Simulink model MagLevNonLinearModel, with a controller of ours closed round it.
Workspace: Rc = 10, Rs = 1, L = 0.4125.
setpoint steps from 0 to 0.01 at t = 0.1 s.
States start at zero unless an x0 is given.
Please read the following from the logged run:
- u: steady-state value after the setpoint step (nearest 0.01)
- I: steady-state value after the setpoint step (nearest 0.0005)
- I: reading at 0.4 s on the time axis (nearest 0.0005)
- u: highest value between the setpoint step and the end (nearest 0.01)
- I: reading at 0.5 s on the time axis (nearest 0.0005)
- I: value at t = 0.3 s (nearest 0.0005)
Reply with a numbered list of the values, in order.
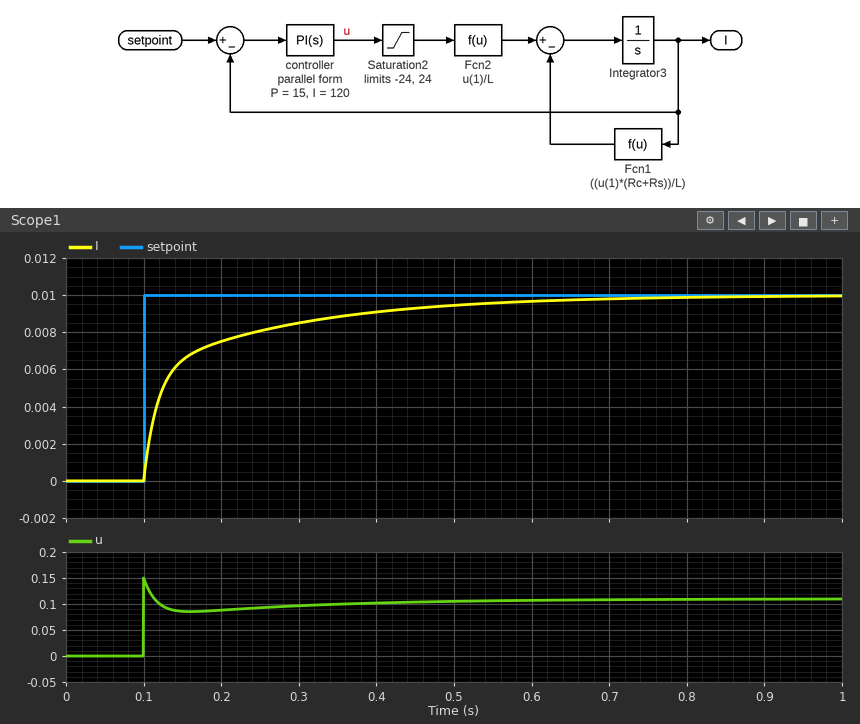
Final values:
1. 0.11
2. 0.0100
3. 0.0090
4. 0.15
5. 0.0095
6. 0.0085
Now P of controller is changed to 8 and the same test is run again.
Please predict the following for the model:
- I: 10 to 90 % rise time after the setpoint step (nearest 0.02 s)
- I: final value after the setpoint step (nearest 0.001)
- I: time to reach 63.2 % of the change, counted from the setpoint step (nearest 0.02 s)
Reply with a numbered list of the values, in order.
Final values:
1. 0.24 s
2. 0.010
3. 0.08 s
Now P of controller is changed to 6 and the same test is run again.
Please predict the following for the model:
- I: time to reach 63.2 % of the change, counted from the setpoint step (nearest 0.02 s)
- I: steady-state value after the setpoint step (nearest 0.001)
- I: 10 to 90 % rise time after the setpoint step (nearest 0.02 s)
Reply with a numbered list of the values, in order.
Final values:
1. 0.08 s
2. 0.010
3. 0.22 s
